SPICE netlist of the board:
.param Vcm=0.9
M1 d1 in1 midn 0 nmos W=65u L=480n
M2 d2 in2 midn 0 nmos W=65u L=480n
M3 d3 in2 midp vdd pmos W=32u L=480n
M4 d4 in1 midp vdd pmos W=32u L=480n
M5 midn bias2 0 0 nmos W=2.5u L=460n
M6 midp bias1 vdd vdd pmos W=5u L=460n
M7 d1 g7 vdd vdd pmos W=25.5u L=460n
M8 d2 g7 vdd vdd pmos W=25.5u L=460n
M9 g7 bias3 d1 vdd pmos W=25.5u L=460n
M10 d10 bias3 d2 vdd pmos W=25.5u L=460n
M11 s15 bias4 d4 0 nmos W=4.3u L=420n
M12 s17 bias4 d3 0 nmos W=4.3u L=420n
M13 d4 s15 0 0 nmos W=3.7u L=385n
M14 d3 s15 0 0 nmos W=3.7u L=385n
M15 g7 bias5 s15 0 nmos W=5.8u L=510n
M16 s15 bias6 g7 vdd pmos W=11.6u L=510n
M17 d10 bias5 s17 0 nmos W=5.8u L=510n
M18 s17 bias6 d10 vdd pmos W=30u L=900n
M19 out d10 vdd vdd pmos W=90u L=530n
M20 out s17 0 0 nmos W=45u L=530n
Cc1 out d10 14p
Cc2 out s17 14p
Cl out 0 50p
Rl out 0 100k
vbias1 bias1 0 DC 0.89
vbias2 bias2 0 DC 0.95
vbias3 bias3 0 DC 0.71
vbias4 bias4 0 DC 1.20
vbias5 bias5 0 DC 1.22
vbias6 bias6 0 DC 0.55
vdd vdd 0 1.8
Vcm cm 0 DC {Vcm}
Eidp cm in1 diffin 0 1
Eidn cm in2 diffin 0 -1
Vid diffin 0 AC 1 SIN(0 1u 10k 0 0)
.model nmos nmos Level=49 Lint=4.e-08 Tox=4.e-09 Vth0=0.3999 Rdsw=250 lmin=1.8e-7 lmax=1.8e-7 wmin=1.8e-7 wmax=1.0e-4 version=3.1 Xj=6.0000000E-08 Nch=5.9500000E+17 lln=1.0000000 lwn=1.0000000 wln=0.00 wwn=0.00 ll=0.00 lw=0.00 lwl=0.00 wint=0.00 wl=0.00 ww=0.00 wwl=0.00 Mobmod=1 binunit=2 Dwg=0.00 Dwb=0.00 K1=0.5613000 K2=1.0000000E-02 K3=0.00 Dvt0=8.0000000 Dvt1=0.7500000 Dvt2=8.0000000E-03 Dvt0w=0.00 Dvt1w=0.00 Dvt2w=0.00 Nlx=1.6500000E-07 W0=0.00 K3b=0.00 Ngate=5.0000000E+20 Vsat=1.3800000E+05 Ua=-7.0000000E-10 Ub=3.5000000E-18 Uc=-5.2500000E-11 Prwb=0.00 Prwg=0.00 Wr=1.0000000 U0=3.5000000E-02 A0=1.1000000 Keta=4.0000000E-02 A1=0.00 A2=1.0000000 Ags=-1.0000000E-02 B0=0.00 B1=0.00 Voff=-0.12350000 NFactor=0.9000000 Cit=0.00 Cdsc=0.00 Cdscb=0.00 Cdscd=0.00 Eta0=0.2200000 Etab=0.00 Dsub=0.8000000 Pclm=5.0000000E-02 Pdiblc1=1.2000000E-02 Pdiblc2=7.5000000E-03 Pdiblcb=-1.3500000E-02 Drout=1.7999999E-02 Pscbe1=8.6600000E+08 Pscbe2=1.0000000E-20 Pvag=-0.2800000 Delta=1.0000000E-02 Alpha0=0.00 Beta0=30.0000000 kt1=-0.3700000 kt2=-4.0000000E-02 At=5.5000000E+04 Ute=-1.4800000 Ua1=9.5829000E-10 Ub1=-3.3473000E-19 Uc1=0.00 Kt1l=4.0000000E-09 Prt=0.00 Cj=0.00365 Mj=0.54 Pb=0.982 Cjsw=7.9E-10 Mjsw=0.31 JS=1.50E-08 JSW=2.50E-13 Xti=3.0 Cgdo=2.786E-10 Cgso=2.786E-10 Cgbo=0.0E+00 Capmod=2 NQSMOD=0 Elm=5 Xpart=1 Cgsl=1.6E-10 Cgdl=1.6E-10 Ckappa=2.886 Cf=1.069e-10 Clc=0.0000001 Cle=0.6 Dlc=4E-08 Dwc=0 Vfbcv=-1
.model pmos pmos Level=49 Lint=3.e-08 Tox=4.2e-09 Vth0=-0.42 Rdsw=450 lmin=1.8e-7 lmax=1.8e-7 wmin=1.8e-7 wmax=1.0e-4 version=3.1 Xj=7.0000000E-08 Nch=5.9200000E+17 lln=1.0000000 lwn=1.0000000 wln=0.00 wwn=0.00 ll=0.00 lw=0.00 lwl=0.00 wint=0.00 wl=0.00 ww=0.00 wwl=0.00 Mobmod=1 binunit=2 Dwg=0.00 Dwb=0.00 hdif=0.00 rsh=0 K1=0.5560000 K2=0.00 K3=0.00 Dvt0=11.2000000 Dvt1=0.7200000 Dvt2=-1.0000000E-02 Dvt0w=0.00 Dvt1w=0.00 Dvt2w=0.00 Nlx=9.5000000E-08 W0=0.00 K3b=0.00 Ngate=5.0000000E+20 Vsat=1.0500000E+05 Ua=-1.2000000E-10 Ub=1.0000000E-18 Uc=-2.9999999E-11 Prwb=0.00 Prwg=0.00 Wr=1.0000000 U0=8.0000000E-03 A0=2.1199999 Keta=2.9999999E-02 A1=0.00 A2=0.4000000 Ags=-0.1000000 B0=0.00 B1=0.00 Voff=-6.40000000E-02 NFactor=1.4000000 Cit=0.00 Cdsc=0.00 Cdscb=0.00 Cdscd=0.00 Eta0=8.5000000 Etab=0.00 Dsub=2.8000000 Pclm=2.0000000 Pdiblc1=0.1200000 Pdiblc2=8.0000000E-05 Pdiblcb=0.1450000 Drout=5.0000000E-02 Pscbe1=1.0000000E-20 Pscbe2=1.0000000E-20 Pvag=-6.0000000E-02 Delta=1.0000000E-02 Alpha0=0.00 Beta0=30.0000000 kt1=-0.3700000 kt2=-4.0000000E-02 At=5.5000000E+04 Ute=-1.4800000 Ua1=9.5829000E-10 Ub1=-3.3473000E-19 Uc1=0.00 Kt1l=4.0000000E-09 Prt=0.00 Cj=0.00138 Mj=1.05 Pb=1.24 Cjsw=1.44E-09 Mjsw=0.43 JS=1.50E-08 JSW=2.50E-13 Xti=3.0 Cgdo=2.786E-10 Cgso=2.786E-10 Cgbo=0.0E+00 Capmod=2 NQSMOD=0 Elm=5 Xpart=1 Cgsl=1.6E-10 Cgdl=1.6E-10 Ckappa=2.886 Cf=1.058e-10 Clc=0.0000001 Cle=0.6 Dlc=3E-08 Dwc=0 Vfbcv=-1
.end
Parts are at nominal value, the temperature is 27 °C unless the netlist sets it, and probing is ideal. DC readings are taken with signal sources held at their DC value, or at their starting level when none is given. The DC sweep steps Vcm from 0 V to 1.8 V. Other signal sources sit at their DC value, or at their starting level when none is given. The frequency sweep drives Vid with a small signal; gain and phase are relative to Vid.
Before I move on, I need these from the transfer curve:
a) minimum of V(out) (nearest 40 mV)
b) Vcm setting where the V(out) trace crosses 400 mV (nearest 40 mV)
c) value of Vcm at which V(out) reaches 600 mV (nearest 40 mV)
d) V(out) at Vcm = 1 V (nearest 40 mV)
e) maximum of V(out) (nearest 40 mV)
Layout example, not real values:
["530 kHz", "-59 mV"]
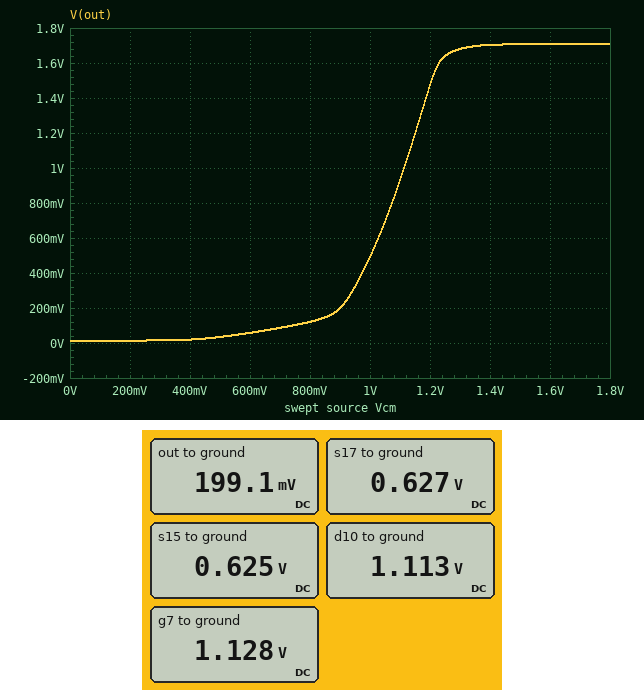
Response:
["0 V", "960 mV", "1.04 V", "480 mV", "1.72 V"]
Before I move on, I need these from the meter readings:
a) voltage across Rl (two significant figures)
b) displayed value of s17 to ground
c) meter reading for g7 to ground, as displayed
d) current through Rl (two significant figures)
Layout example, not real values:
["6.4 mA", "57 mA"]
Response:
["200 mV", "0.627 V", "1.128 V", "2.0 µA"]
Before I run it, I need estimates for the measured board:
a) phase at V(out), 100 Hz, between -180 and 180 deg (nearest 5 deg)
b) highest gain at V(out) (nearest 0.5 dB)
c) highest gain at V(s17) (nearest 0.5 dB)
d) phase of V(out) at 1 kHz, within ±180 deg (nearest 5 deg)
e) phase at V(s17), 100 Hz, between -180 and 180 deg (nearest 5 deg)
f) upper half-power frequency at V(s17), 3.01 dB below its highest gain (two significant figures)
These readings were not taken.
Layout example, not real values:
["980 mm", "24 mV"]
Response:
["-20 deg", "92.0 dB", "55.5 dB", "-75 deg", "160 deg", "270 Hz"]
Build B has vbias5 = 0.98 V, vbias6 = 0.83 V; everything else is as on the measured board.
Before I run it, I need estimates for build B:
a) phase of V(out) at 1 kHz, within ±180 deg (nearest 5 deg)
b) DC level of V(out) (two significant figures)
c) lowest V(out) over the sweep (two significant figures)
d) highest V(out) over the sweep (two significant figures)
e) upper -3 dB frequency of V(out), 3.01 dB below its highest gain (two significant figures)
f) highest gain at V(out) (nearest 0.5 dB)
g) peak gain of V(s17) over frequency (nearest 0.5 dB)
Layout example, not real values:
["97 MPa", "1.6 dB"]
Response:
["-50 deg", "120 mV", "1.0 mV", "1.8 V", "680 Hz", "55.0 dB", "36.5 dB"]
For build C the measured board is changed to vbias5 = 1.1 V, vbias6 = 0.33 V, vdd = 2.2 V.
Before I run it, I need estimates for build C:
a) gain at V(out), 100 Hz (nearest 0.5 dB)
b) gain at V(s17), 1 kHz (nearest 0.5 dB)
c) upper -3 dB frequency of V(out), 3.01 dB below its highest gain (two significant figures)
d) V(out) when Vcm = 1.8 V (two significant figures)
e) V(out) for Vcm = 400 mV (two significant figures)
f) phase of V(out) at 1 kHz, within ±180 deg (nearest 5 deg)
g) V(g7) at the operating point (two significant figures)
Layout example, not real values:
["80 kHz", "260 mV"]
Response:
["48.0 dB", "64.0 dB", "18 kHz", "60 mV", "65 mV", "-5 deg", "1.4 V"]
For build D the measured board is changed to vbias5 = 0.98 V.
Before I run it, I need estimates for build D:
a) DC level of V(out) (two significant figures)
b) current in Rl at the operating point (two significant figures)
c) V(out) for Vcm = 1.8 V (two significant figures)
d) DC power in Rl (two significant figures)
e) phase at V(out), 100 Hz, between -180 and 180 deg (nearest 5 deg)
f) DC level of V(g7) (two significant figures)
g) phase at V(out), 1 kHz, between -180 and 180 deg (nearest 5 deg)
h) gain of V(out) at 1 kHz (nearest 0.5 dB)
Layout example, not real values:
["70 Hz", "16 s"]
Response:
["430 mV", "4.3 µA", "1.8 V", "1.8 µW", "-5 deg", "1.1 V", "-45 deg", "71.5 dB"]
